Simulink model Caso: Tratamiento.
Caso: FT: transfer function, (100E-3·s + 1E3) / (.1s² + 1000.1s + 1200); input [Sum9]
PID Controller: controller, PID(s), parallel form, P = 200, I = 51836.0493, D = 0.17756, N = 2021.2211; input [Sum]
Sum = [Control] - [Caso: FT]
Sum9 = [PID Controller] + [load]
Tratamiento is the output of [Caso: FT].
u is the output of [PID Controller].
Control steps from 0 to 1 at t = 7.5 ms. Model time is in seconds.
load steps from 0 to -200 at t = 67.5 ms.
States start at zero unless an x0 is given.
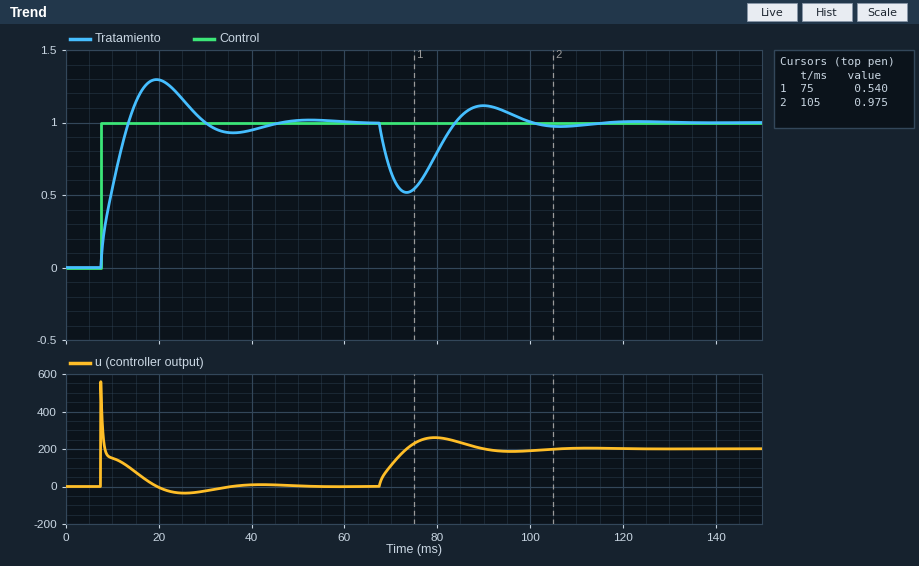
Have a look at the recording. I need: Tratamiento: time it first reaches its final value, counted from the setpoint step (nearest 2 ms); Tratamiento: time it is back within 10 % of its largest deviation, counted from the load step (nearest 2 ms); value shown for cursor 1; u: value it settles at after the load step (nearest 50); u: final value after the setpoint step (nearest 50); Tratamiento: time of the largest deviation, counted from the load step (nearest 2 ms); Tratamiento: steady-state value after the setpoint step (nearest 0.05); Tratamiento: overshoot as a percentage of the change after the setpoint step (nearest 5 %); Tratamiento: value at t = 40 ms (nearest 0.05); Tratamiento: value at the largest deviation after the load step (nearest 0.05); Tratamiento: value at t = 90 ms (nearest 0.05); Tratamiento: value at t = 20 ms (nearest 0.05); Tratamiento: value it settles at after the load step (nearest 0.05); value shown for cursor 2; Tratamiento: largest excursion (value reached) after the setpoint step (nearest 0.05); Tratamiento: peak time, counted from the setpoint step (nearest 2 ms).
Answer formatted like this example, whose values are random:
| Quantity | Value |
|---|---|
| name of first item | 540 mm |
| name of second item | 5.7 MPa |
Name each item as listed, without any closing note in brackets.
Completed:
| Quantity | Value |
|---|---|
| Tratamiento: time it first reaches its final value, counted from the setpoint step | 6 ms |
| Tratamiento: time it is back within 10 % of its largest deviation, counted from the load step | 30 ms |
| value shown for cursor 1 | 0.540 |
| u: value it settles at after the load step | 200 |
| u: final value after the setpoint step | 0 |
| Tratamiento: time of the largest deviation, counted from the load step | 6 ms |
| Tratamiento: steady-state value after the setpoint step | 1.00 |
| Tratamiento: overshoot as a percentage of the change after the setpoint step | 30 % |
| Tratamiento: value at t = 40 ms | 0.95 |
| Tratamiento: value at the largest deviation after the load step | 0.50 |
| Tratamiento: value at t = 90 ms | 1.10 |
| Tratamiento: value at t = 20 ms | 1.30 |
| Tratamiento: value it settles at after the load step | 1.00 |
| value shown for cursor 2 | 0.975 |
| Tratamiento: largest excursion (value reached) after the setpoint step | 1.30 |
| Tratamiento: peak time, counted from the setpoint step | 12 ms |
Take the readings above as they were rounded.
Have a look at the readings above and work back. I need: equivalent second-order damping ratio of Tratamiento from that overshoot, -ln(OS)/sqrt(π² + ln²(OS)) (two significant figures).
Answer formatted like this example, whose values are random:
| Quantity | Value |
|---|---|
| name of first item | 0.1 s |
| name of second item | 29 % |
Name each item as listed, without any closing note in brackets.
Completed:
| Quantity | Value |
|---|---|
| equivalent second-order damping ratio of Tratamiento from that overshoot, -ln(OS)/sqrt(π² + ln²(OS)) | 0.36 |
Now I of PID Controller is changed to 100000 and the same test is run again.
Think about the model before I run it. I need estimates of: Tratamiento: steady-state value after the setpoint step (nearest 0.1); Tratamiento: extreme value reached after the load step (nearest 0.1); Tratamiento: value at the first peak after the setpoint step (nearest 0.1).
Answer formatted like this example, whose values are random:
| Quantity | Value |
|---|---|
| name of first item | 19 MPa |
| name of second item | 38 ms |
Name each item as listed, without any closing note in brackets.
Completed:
| Quantity | Value |
|---|---|
| Tratamiento: steady-state value after the setpoint step | 1.0 |
| Tratamiento: extreme value reached after the load step | 0.6 |
| Tratamiento: value at the first peak after the setpoint step | 1.4 |
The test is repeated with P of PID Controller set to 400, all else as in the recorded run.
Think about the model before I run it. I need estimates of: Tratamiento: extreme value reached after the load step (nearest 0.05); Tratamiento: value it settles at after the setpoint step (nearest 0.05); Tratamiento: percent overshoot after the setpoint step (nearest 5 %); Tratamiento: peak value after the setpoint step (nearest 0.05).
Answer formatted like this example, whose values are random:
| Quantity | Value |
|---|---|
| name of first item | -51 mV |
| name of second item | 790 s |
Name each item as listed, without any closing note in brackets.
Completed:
| Quantity | Value |
|---|---|
| Tratamiento: extreme value reached after the load step | 0.65 |
| Tratamiento: value it settles at after the setpoint step | 1.00 |
| Tratamiento: percent overshoot after the setpoint step | 15 % |
| Tratamiento: peak value after the setpoint step | 1.15 |
